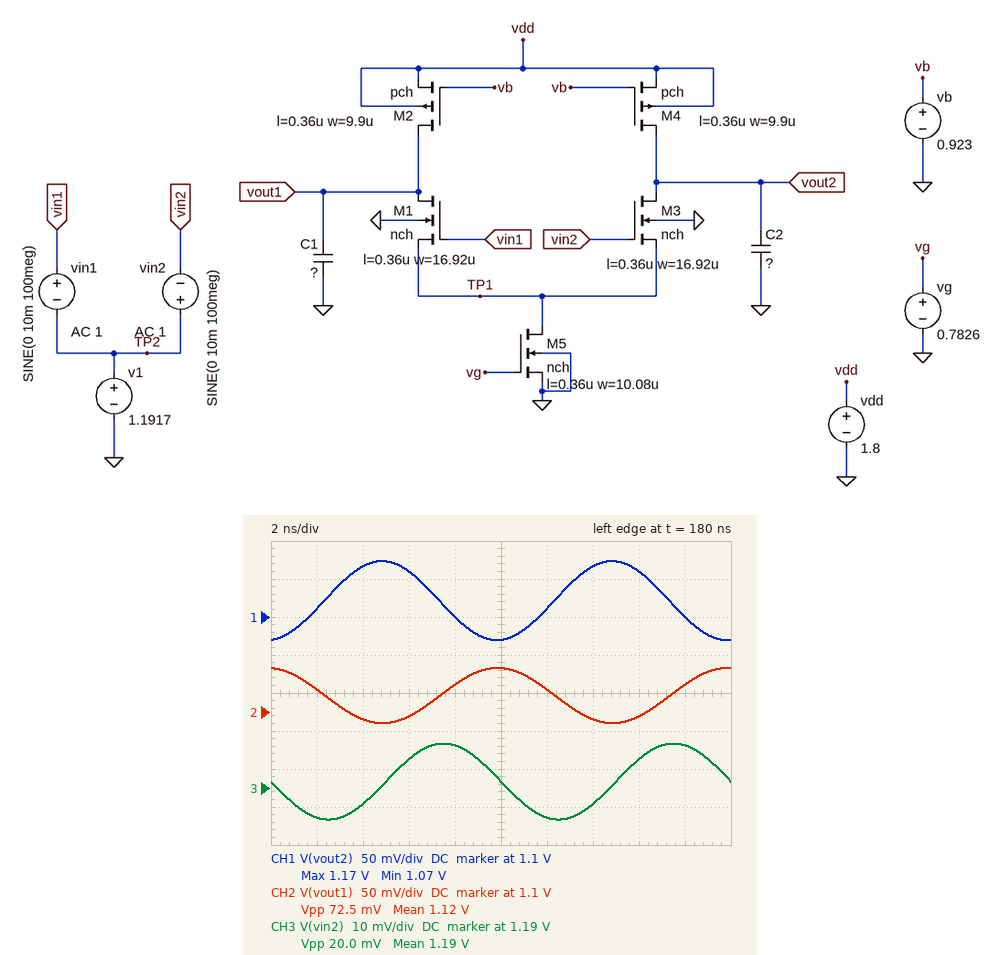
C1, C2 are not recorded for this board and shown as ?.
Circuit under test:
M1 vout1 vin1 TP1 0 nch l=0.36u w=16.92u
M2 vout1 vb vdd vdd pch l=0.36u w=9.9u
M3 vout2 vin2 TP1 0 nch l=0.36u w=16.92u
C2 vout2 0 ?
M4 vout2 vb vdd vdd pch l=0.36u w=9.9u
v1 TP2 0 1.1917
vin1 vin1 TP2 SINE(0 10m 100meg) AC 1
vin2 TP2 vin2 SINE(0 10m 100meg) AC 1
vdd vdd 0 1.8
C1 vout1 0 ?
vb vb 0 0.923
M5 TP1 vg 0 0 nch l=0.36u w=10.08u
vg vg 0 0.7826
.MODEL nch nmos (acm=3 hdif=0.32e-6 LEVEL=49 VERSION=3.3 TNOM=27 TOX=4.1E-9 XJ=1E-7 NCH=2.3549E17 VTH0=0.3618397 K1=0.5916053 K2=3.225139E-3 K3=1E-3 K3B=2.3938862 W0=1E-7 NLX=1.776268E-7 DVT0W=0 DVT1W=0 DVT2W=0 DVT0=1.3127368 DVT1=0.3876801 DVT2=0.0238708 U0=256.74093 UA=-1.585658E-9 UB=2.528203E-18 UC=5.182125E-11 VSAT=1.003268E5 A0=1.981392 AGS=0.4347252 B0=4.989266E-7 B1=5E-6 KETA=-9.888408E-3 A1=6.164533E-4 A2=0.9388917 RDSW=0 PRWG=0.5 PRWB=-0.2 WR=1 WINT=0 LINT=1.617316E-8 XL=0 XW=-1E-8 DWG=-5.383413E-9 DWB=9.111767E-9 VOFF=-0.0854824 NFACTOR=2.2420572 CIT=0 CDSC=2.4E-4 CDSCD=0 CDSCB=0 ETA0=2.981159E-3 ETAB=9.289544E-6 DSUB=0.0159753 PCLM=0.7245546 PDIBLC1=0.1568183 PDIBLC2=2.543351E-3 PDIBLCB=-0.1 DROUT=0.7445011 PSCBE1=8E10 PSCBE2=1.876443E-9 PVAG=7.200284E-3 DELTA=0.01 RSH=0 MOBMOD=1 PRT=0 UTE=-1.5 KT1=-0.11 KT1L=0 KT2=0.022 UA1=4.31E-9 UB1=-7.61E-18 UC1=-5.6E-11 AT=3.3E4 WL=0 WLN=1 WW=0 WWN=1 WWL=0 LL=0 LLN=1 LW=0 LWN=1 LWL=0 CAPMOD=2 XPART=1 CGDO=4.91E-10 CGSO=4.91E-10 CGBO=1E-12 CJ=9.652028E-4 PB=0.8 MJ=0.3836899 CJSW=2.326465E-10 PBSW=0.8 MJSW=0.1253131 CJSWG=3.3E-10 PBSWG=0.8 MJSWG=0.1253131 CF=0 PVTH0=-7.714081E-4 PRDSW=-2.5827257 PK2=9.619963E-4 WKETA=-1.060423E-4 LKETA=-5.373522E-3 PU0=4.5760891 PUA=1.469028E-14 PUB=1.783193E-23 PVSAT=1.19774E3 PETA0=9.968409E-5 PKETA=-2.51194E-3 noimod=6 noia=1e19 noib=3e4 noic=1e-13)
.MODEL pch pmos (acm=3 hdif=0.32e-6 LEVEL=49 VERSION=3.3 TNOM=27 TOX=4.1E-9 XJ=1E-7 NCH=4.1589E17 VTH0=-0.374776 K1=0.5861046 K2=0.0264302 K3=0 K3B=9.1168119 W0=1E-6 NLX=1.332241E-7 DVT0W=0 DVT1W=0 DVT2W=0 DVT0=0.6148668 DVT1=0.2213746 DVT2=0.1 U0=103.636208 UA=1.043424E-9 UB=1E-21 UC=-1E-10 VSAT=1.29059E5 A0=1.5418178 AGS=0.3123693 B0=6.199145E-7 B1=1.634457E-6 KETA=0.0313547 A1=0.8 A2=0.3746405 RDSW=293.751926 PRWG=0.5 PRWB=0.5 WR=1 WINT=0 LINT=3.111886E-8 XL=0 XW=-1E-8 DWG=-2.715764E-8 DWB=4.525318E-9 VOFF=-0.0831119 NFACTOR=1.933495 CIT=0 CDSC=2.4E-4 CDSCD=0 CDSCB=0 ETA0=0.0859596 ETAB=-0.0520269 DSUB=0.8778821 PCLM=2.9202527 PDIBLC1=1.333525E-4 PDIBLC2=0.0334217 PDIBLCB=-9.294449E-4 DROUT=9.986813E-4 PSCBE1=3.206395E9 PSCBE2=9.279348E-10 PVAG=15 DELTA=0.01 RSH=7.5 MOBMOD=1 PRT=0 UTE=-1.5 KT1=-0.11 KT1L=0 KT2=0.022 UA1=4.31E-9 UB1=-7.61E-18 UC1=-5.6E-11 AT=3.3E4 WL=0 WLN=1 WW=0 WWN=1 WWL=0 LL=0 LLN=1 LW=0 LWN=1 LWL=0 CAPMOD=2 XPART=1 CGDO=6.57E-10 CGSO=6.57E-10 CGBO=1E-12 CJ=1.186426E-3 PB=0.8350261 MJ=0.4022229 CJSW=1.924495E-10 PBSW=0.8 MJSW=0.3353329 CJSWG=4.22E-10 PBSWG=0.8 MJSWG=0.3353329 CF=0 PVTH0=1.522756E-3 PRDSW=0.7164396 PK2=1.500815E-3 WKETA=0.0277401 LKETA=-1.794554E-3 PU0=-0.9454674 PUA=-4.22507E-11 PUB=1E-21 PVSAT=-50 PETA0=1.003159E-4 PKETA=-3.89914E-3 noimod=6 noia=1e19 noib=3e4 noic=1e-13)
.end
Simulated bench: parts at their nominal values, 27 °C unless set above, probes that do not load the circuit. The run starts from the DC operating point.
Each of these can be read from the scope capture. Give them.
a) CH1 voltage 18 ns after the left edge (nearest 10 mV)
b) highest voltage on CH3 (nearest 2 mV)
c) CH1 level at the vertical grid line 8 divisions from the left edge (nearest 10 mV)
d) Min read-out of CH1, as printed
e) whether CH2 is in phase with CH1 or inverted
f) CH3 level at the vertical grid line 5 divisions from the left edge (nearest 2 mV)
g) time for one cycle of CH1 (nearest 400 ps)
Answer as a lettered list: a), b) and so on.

a) 1.10 V
b) 1.202 V
c) 1.16 V
d) 1.07 V
e) inverted
f) 1.192 V
g) 10.0 ns
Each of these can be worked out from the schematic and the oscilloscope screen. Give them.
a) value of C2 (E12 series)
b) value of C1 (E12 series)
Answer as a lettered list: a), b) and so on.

a) 560 fF
b) 820 fF
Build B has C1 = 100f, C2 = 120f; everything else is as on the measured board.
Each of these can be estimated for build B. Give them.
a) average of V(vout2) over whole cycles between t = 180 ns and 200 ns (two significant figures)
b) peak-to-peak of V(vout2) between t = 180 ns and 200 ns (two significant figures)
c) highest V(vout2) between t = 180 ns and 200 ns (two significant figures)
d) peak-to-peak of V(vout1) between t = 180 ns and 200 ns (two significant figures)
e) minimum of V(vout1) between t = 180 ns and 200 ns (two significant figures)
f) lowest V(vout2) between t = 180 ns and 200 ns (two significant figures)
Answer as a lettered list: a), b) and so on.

a) 1.1 V
b) 350 mV
c) 1.3 V
d) 390 mV
e) 910 mV
f) 940 mV
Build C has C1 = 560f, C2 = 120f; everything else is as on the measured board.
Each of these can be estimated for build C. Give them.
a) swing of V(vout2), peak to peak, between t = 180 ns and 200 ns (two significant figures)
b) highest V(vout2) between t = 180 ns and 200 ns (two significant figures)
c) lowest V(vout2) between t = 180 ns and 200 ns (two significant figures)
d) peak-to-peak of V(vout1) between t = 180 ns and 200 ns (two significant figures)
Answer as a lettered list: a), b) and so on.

a) 360 mV
b) 1.3 V
c) 930 mV
d) 100 mV
